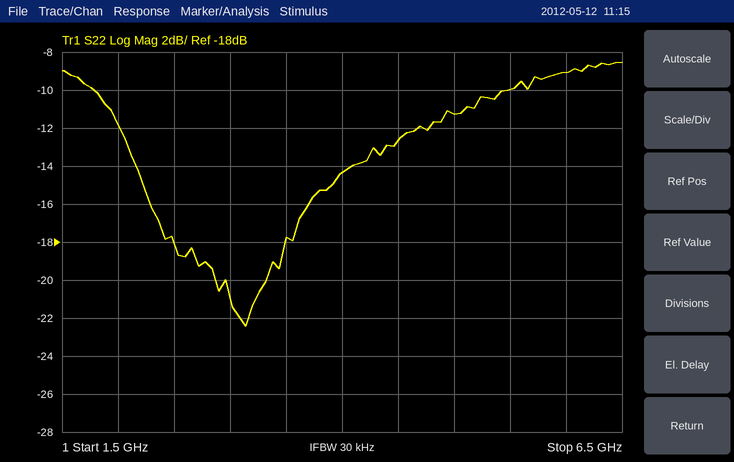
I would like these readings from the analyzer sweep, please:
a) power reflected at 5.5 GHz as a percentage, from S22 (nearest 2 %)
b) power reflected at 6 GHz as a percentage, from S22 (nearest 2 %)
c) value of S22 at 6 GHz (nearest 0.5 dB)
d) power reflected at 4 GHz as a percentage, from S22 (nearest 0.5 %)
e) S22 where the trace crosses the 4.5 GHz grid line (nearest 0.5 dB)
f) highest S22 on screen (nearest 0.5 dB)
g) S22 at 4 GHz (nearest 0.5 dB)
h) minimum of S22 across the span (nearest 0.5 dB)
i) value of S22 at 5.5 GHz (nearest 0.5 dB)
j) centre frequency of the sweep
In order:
10 %
12 %
-9.0 dB
3.5 %
-12.5 dB
-8.5 dB
-14.5 dB
-22.5 dB
-10.0 dB
4 GHz
